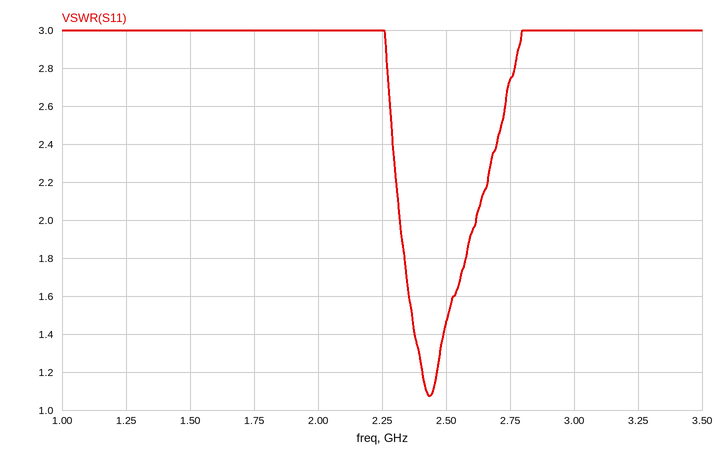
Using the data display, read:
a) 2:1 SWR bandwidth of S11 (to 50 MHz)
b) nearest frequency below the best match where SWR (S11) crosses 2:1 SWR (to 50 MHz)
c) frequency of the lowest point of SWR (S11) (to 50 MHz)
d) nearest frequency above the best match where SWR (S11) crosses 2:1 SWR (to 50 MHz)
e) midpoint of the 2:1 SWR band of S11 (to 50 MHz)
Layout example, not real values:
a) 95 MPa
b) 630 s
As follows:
a) 300 MHz
b) 2.30 GHz
c) 2.45 GHz
d) 2.60 GHz
e) 2.45 GHz
